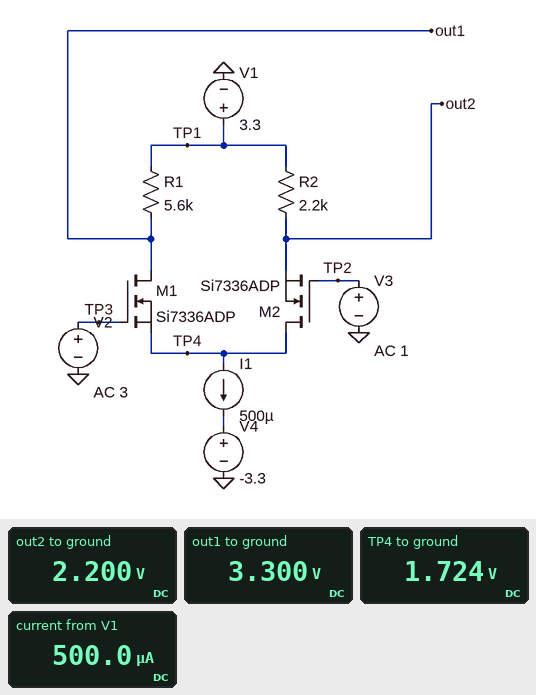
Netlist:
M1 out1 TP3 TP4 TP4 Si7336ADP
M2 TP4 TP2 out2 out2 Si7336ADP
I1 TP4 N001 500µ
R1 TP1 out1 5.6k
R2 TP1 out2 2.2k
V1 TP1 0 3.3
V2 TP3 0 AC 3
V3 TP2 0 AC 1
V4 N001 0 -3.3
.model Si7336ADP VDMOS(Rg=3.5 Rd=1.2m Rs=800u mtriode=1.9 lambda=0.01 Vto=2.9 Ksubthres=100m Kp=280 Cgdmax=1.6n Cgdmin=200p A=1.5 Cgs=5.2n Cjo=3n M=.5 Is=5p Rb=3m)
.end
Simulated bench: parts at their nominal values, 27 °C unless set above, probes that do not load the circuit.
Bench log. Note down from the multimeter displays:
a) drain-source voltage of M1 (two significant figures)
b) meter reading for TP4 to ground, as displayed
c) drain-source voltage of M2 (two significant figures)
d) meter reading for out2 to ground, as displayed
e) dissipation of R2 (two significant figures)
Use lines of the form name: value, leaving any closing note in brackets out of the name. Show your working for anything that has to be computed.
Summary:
drain-source voltage of M1: 3.3 V - 1.724 V = 1.6 V
meter reading for TP4 to ground, as displayed: 1.724 V
drain-source voltage of M2: 1.724 V - 2.2 V = -480 mV
meter reading for out2 to ground, as displayed: 2.200 V
dissipation of R2: (3.3 V - 2.2 V)^2 / 2.2 kΩ = 550 µW
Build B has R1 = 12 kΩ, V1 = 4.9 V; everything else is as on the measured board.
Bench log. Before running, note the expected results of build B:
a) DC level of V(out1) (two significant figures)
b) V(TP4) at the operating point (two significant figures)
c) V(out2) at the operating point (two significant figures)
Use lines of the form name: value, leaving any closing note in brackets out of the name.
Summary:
DC level of V(out1): 4.9 V
V(TP4) at the operating point: 3.3 V
V(out2) at the operating point: 3.8 V
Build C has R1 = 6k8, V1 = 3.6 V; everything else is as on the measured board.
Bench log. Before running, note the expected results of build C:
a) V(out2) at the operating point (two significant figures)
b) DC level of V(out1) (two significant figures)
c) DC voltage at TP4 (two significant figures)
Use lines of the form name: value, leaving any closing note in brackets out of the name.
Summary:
V(out2) at the operating point: 2.5 V
DC level of V(out1): 3.6 V
DC voltage at TP4: 2.0 V
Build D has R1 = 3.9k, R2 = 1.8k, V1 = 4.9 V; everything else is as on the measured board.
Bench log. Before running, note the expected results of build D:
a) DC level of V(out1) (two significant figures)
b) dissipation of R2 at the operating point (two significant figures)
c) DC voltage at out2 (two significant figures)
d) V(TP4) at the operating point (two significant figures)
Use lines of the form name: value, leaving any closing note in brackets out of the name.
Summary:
DC level of V(out1): 4.9 V
dissipation of R2 at the operating point: 450 µW
DC voltage at out2: 4.0 V
V(TP4) at the operating point: 3.5 V
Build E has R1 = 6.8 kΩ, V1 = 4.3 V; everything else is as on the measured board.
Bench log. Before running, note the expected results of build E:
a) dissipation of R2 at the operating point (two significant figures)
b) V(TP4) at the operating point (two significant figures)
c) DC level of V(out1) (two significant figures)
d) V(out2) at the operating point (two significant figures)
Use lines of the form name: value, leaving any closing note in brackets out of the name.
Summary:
dissipation of R2 at the operating point: 550 µW
V(TP4) at the operating point: 2.7 V
DC level of V(out1): 4.3 V
V(out2) at the operating point: 3.2 V
